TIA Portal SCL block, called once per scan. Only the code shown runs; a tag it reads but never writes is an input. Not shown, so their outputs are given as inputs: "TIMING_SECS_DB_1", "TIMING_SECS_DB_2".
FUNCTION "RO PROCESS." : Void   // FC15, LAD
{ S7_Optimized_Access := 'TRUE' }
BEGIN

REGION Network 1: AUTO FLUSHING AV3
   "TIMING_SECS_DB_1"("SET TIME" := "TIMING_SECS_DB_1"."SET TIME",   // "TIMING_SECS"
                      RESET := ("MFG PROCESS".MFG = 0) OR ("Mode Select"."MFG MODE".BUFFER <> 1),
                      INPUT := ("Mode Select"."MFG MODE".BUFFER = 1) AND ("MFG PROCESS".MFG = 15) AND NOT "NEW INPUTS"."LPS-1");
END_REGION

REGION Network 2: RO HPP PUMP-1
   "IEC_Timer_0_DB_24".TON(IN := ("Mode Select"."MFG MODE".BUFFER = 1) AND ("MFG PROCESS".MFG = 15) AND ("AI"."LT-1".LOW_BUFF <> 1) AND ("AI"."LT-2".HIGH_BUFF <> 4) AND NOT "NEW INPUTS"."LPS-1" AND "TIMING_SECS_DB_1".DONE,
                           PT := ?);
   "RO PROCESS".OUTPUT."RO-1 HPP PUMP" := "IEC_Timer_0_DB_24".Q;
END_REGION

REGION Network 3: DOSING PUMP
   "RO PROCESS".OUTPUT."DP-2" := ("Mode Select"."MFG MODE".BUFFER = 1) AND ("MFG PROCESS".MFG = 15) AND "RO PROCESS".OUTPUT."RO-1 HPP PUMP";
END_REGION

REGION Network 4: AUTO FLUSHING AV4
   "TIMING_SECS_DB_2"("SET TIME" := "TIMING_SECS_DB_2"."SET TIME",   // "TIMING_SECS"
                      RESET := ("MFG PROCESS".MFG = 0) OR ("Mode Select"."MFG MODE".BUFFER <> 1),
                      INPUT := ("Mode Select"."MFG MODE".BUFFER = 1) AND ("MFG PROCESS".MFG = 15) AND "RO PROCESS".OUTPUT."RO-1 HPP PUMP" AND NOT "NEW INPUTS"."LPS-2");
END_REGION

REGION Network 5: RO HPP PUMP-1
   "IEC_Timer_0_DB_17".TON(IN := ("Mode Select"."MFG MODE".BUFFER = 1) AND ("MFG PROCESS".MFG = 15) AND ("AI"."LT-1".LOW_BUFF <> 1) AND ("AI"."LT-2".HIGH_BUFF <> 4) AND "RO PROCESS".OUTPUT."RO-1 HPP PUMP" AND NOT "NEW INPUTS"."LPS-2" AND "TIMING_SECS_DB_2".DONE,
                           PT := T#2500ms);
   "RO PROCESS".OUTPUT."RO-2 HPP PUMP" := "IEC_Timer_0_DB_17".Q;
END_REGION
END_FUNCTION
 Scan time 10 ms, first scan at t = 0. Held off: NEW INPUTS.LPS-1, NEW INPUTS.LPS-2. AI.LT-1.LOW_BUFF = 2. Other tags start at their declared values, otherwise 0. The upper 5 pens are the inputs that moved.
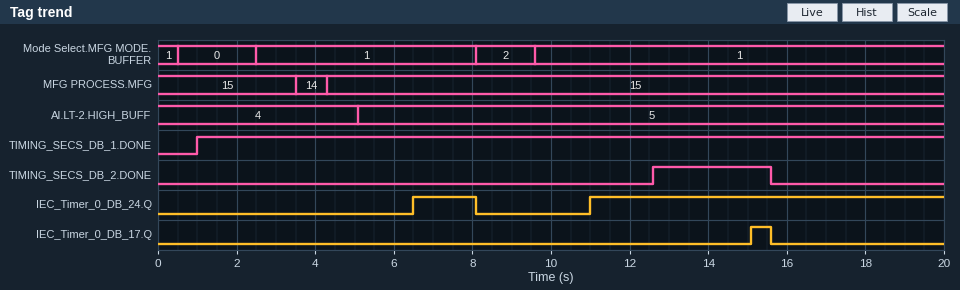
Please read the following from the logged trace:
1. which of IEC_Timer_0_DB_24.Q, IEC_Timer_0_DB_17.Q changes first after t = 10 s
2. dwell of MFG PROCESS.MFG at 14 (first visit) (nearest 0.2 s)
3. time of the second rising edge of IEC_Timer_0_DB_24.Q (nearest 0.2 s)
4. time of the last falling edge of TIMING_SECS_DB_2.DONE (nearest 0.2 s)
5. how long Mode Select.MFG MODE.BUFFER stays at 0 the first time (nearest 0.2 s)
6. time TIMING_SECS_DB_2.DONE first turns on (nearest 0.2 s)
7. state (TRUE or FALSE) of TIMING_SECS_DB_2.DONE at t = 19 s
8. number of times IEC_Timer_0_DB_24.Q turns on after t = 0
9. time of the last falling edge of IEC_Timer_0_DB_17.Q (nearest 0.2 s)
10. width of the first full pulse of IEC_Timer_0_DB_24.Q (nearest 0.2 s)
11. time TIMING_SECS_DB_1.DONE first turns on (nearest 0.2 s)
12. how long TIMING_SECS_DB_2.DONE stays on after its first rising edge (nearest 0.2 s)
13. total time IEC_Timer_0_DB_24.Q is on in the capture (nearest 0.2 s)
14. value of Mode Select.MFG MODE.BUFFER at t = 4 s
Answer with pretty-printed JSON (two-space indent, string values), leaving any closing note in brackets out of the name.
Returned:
{
  "which of IEC_Timer_0_DB_24.Q, IEC_Timer_0_DB_17.Q changes first after t = 10 s": "IEC_Timer_0_DB_24.Q",
  "dwell of MFG PROCESS.MFG at 14 (first visit)": "0.8 s",
  "time of the second rising edge of IEC_Timer_0_DB_24.Q": "11.0 s",
  "time of the last falling edge of TIMING_SECS_DB_2.DONE": "15.6 s",
  "how long Mode Select.MFG MODE.BUFFER stays at 0 the first time": "2.0 s",
  "time TIMING_SECS_DB_2.DONE first turns on": "12.6 s",
  "state (TRUE or FALSE) of TIMING_SECS_DB_2.DONE at t = 19 s": "FALSE",
  "number of times IEC_Timer_0_DB_24.Q turns on after t = 0": "2",
  "time of the last falling edge of IEC_Timer_0_DB_17.Q": "15.6 s",
  "width of the first full pulse of IEC_Timer_0_DB_24.Q": "1.6 s",
  "time TIMING_SECS_DB_1.DONE first turns on": "1.0 s",
  "how long TIMING_SECS_DB_2.DONE stays on after its first rising edge": "3.0 s",
  "total time IEC_Timer_0_DB_24.Q is on in the capture": "10.6 s",
  "value of Mode Select.MFG MODE.BUFFER at t = 4 s": "1"
}
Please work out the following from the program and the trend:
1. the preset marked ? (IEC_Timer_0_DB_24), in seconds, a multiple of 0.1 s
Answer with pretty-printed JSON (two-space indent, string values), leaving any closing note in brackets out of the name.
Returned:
{
  "the preset marked ? (IEC_Timer_0_DB_24), in seconds, a multiple of 0.1 s": "1.4 s"
}
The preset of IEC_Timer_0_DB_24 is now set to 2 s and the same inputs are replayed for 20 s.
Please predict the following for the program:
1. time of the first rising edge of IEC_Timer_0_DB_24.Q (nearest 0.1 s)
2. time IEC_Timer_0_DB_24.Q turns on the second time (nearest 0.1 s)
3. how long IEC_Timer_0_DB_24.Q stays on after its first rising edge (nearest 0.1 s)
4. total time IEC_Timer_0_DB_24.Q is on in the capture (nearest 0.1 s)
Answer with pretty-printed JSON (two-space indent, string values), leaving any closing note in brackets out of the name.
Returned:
{
  "time of the first rising edge of IEC_Timer_0_DB_24.Q": "7.1 s",
  "time IEC_Timer_0_DB_24.Q turns on the second time": "11.6 s",
  "how long IEC_Timer_0_DB_24.Q stays on after its first rising edge": "1.0 s",
  "total time IEC_Timer_0_DB_24.Q is on in the capture": "9.4 s"
}
